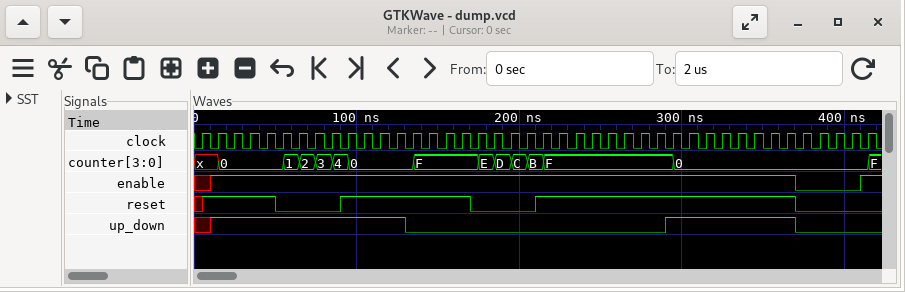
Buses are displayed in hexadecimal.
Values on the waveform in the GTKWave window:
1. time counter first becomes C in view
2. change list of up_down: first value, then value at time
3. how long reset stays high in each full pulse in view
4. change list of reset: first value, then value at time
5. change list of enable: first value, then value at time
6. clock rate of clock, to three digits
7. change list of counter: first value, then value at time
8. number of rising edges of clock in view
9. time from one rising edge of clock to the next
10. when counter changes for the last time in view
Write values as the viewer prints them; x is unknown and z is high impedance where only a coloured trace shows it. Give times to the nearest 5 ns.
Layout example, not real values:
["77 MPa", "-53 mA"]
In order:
["195 ns", "x, 1 at 10 ns, 0 at 130 ns, 1 at 290 ns, 0 at 370 ns", "80 ns, 160 ns", "x, 1 at 5 ns, 0 at 50 ns, 1 at 90 ns, 0 at 170 ns, 1 at 210 ns, 0 at 370 ns", "x, 1 at 10 ns, 0 at 370 ns, 1 at 410 ns", "100 MHz", "x, 0 at 15 ns, 1 at 55 ns, 2 at 65 ns, 3 at 75 ns, 4 at 85 ns, 0 at 95 ns, F at 135 ns, E at 175 ns, D at 185 ns, C at 195 ns, B at 205 ns, F at 215 ns, 0 at 295 ns, F at 415 ns", "42", "10 ns", "415 ns"]
